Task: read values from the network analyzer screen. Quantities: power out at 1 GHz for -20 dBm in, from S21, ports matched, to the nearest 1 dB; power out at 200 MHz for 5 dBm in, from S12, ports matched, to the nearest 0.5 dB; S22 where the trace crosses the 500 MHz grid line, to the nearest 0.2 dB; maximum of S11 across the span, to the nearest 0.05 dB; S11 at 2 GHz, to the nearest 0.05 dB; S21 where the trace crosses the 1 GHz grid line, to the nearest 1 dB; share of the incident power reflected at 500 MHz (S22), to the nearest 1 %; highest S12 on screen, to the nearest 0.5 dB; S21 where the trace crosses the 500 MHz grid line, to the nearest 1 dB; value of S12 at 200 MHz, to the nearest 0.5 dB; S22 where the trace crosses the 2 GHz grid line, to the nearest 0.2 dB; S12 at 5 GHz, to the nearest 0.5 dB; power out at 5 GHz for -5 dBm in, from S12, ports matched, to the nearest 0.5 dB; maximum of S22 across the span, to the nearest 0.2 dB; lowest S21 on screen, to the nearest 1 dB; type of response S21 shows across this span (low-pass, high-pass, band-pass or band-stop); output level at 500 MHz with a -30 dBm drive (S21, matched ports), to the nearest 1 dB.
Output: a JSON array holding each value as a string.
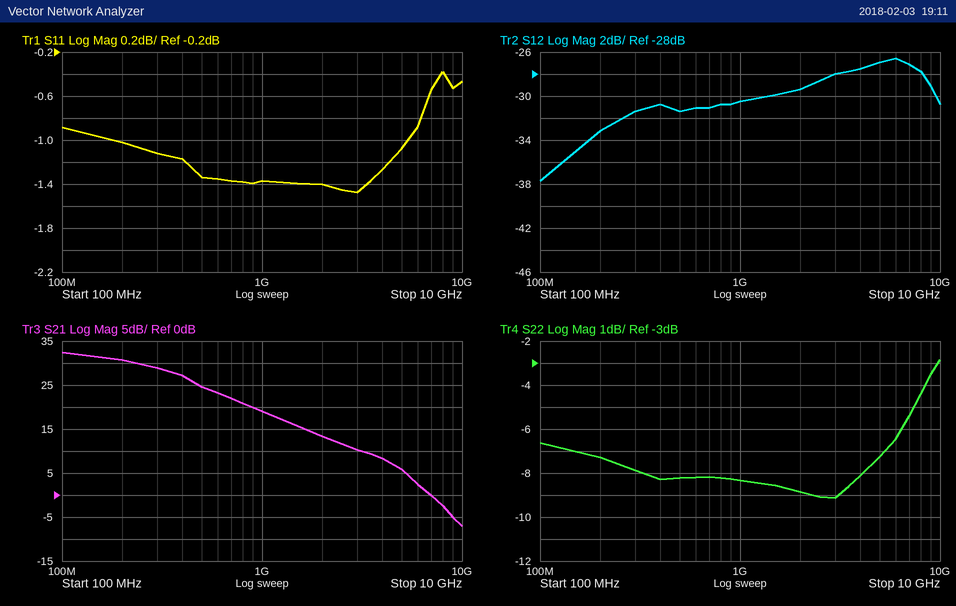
["-1 dBm", "-28.0 dBm", "-8.2 dB", "-0.40 dB", "-1.40 dB", "19 dB", "15 %", "-26.5 dB", "25 dB", "-33.0 dB", "-8.8 dB", "-27.0 dB", "-32.0 dBm", "-2.8 dB", "-7 dB", "low-pass", "-5 dBm"]
